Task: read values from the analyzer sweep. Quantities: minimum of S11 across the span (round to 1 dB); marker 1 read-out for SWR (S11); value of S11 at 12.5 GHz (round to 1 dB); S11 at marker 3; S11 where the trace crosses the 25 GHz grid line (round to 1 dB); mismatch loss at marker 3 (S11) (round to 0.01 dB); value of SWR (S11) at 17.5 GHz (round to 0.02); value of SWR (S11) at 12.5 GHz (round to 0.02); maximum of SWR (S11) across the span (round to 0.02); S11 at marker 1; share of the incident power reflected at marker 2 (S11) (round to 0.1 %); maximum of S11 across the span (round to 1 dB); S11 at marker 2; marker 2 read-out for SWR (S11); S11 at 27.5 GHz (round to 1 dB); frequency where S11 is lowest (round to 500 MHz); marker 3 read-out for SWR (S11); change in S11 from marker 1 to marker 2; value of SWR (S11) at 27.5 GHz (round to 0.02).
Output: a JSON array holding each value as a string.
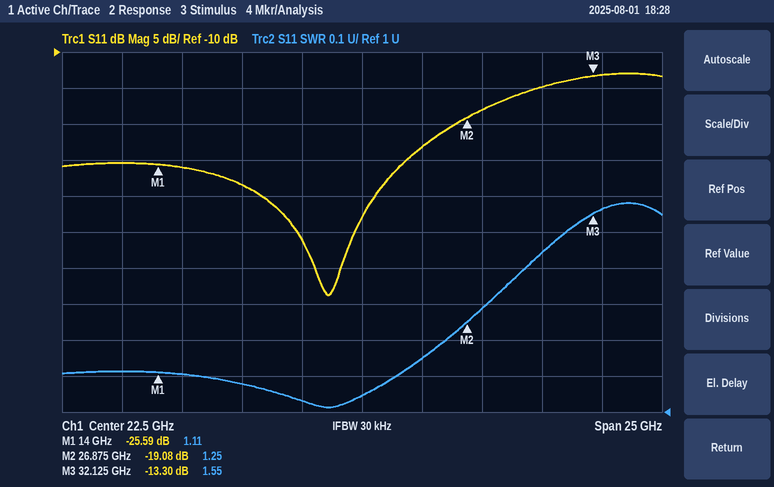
["-44 dB", "1.11", "-25 dB", "-13.30 dB", "-23 dB", "0.21 dB", "1.08", "1.12", "1.58", "-25.59 dB", "1.2 %", "-13 dB", "-19.08 dB", "1.25", "-18 dB", "21.0 GHz", "1.55", "6.51 dB", "1.28"]
